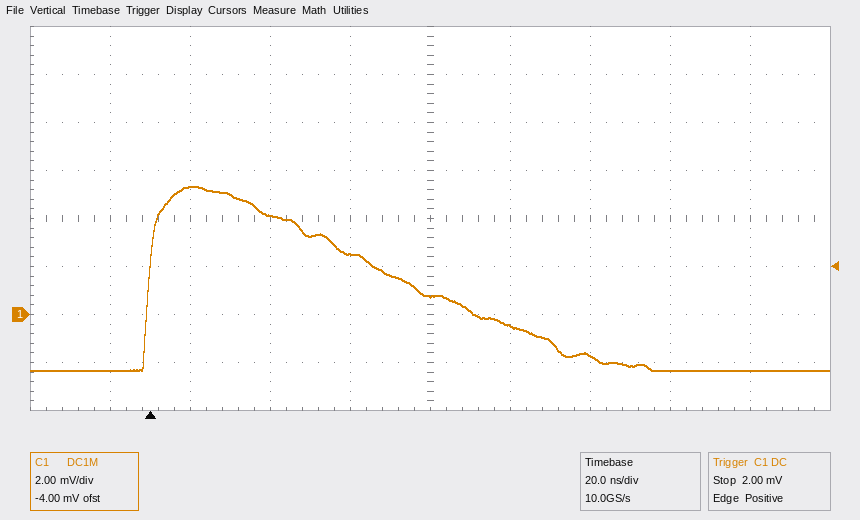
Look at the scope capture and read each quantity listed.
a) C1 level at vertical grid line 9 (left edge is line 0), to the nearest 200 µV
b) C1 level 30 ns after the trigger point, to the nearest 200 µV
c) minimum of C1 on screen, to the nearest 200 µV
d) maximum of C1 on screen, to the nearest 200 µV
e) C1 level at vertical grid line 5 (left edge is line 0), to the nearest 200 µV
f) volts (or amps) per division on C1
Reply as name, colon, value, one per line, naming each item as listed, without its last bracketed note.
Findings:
C1 level at vertical grid line 9 (left edge is line 0), to the nearest 200 µV: -2.4 mV
C1 level 30 ns after the trigger point, to the nearest 200 µV: 4.2 mV
minimum of C1 on screen, to the nearest 200 µV: -2.4 mV
maximum of C1 on screen, to the nearest 200 µV: 5.4 mV
C1 level at vertical grid line 5 (left edge is line 0), to the nearest 200 µV: 800 µV
volts (or amps) per division on C1: 2 mV
